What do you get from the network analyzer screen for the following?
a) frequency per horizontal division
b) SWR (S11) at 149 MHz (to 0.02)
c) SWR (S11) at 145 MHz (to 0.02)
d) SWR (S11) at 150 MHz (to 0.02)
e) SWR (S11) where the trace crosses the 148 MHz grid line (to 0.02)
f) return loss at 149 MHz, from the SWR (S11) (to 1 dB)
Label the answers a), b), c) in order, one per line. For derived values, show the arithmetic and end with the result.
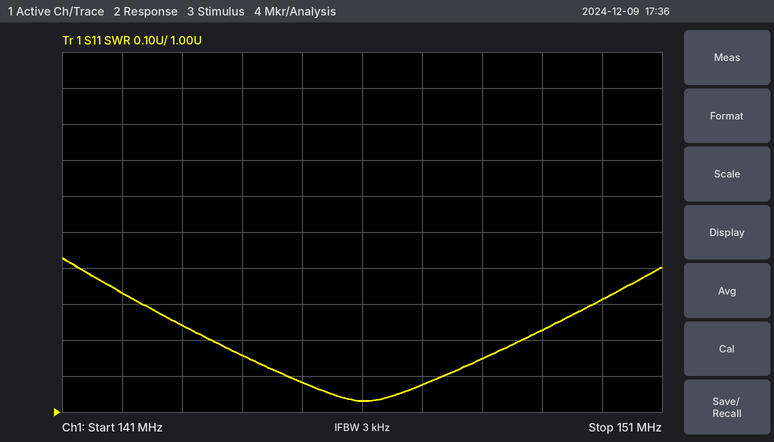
a) 1 MHz
b) 1.22
c) 1.08
d) 1.32
e) 1.14
f) −20 log10((1.22 − 1)/(1.22 + 1)) ≈ 20 dB
